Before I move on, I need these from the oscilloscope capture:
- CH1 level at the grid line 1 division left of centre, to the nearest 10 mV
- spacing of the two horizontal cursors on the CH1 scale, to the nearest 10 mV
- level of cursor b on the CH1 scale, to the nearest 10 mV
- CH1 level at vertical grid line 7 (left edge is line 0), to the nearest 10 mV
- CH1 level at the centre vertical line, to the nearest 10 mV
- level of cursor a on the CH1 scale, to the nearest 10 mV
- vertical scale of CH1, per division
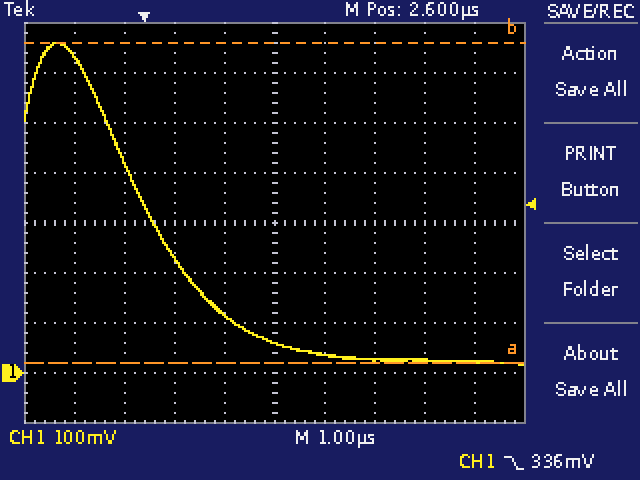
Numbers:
120 mV
640 mV
660 mV
30 mV
60 mV
20 mV
100 mV
